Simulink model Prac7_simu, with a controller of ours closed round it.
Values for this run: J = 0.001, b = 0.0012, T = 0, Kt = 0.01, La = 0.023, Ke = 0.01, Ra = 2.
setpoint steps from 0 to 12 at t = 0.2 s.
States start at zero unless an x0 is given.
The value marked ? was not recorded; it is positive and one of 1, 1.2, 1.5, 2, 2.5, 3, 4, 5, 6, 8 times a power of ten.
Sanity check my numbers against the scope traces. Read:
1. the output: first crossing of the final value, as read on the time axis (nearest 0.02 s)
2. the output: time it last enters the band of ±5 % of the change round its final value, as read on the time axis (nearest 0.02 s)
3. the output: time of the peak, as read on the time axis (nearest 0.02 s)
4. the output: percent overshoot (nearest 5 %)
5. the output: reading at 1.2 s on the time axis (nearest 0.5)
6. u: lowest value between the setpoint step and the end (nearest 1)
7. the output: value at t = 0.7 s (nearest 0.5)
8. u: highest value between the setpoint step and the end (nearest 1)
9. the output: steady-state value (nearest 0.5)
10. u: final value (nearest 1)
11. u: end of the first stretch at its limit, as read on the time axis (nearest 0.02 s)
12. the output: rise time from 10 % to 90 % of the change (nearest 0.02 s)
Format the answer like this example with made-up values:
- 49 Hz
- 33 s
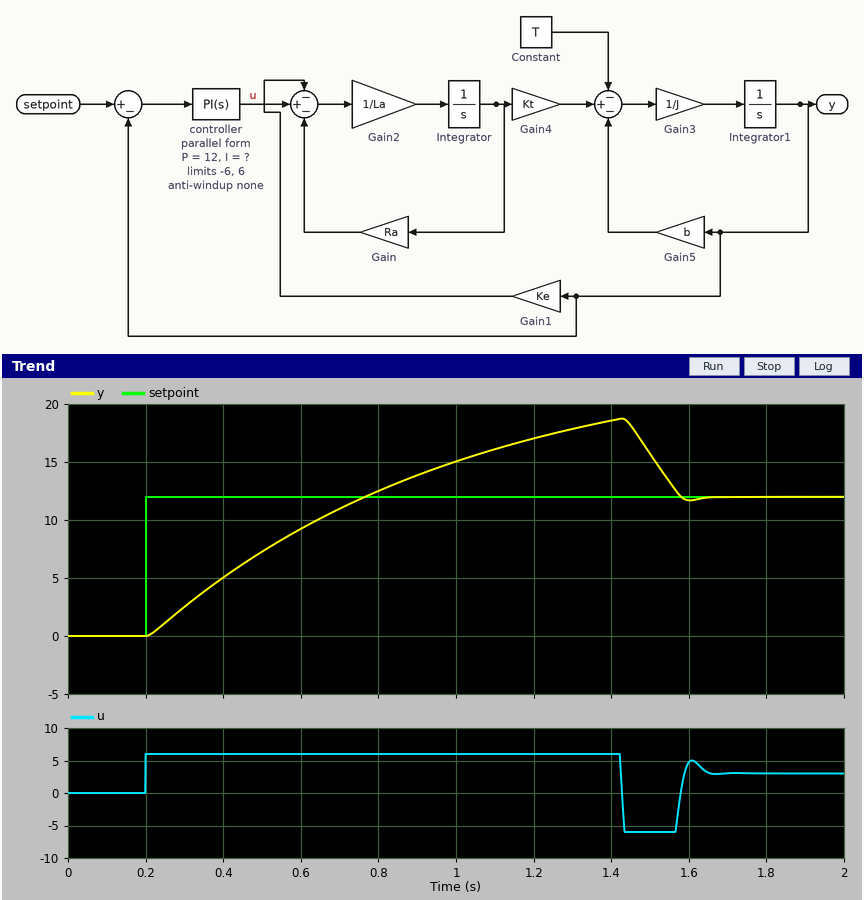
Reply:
- 0.76 s
- 1.56 s
- 1.42 s
- 55 %
- 17.0
- -6
- 11.0
- 6
- 12.0
- 3
- 1.42 s
- 0.44 s
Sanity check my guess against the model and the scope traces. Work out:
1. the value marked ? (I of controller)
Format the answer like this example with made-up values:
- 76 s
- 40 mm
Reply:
- 150
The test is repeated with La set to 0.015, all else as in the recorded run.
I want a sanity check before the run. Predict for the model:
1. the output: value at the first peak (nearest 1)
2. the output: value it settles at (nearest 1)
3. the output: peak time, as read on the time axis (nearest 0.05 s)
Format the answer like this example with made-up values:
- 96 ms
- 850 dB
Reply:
- 19
- 12
- 1.40 s
